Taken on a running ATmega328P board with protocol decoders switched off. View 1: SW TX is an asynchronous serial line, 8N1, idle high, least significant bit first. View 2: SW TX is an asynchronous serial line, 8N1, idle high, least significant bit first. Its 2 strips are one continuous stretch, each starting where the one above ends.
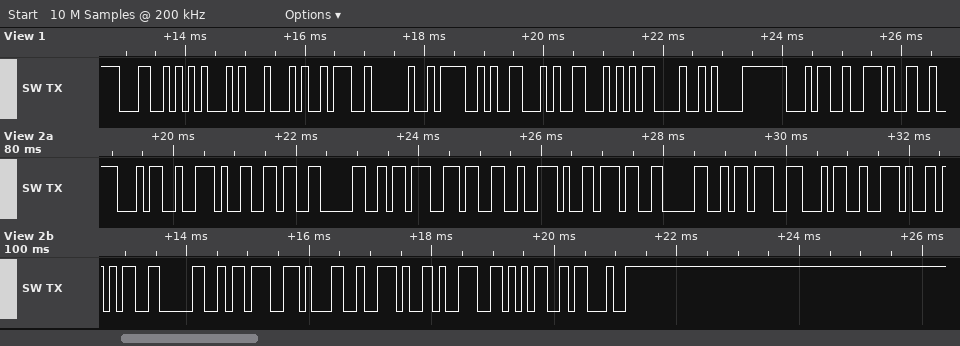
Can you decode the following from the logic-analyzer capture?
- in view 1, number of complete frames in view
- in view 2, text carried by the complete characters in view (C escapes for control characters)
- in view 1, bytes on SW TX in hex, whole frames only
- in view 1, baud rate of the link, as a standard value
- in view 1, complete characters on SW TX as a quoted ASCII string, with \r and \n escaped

12
"4.60;3.70;4.50;1.95#"
4C 45 44 3A 20 4F 46 46 0D 0A 34 2E
9600 baud
"LED: OFF\r\n4."
